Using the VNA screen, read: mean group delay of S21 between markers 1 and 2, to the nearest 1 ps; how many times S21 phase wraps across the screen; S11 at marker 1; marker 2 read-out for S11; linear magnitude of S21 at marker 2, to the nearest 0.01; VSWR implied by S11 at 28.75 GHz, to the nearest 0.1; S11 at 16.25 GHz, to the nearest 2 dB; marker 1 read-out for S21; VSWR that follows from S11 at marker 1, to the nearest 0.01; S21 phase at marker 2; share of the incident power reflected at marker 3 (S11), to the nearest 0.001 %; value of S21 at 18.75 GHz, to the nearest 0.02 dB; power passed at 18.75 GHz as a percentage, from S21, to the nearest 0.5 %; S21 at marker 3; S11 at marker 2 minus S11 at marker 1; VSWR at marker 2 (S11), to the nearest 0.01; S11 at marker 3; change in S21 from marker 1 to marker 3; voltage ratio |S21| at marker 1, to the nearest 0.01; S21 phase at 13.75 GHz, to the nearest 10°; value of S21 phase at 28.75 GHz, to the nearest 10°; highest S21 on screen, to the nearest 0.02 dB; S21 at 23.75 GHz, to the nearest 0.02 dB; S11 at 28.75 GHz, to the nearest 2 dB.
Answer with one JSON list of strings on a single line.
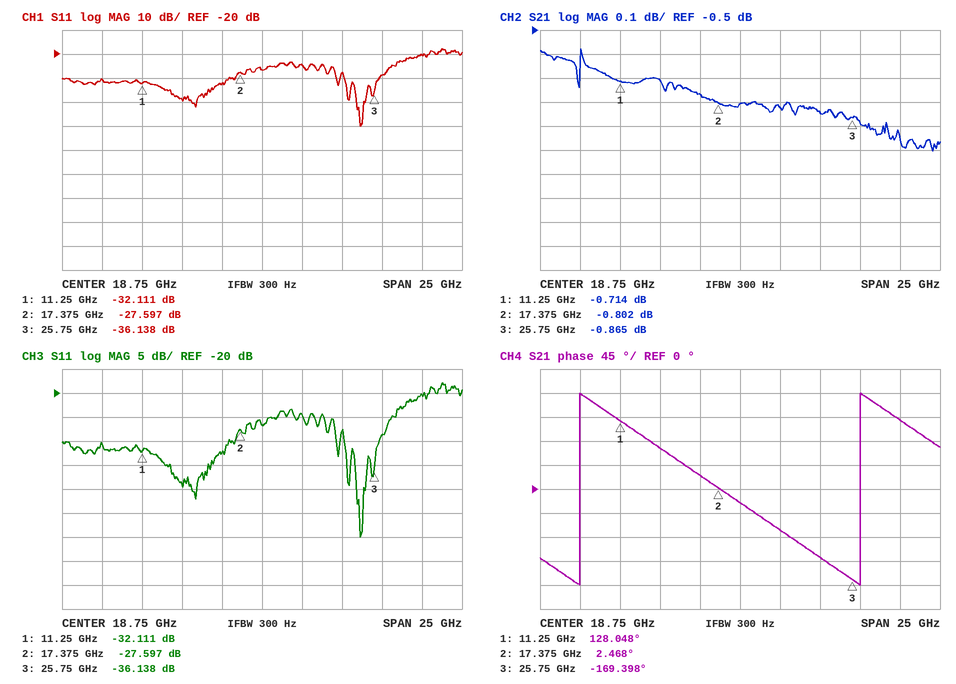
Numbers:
["57 ps", "2", "-32.111 dB", "-27.597 dB", "0.91", "1.2", "-32 dB", "-0.714 dB", "1.05", "2.468°", "0.024 %", "-0.80 dB", "83.0 %", "-0.865 dB", "4.514 dB", "1.09", "-36.138 dB", "-0.151 dB", "0.92", "80°", "130°", "-0.58 dB", "-0.84 dB", "-20 dB"]
